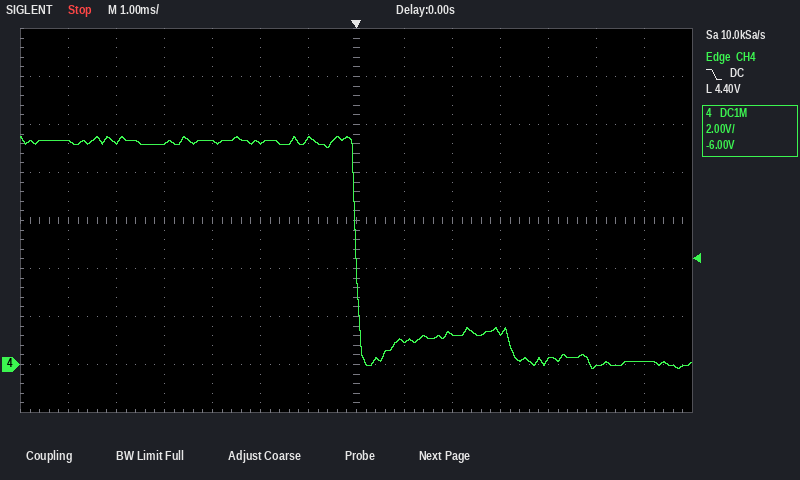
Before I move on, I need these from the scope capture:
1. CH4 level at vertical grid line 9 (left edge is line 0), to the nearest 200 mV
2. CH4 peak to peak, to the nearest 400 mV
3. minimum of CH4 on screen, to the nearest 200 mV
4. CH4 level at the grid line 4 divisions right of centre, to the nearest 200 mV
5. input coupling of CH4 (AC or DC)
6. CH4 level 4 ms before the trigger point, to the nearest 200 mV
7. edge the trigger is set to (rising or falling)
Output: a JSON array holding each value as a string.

["1.2 V", "9.6 V", "-200 mV", "200 mV", "DC", "9.2 V", "falling"]
